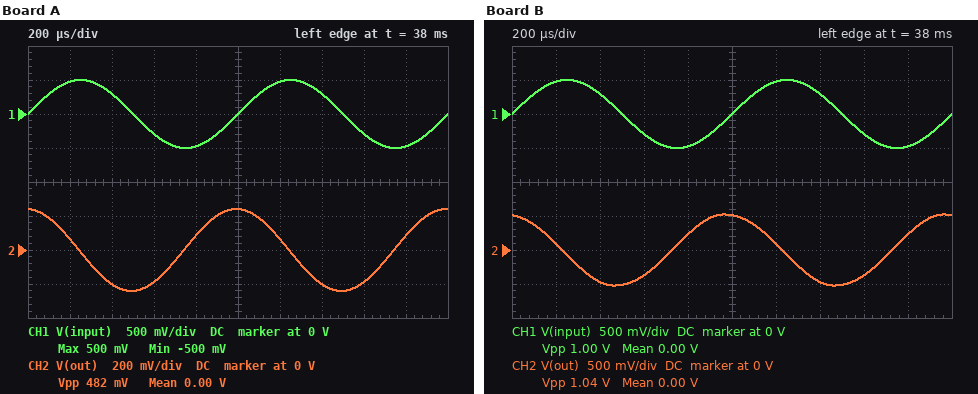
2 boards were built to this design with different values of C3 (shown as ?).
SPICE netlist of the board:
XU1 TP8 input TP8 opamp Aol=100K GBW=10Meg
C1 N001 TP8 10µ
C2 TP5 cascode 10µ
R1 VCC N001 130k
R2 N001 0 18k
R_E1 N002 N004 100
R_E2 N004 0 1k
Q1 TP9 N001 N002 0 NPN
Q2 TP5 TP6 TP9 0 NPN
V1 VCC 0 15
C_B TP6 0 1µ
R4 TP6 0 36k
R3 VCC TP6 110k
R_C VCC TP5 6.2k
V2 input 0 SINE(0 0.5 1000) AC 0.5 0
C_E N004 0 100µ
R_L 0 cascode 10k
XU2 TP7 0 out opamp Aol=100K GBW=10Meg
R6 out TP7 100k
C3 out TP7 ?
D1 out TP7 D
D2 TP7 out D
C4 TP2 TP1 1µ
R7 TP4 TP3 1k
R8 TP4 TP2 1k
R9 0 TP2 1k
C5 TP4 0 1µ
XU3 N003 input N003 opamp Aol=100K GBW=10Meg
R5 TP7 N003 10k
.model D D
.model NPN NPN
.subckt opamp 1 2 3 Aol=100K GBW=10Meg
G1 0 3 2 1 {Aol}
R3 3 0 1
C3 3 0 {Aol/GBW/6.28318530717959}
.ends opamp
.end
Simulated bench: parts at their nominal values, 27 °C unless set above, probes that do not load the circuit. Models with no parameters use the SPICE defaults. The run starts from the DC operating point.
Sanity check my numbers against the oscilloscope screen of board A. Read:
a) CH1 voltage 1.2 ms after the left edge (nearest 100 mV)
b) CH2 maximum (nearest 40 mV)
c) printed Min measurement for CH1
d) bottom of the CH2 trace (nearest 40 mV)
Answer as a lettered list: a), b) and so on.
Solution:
a) 500 mV
b) 240 mV
c) -500 mV
d) -240 mV
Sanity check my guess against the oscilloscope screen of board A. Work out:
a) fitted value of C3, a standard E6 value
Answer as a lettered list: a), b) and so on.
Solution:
a) 33 nF
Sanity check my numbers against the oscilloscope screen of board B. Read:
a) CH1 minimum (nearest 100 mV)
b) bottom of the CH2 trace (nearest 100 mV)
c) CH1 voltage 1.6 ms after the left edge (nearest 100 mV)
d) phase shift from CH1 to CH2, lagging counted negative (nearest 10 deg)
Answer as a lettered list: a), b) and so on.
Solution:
a) -500 mV
b) -500 mV
c) -300 mV
d) 100 deg
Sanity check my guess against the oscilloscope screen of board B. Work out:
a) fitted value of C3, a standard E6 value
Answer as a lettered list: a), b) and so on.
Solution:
a) 15 nF
